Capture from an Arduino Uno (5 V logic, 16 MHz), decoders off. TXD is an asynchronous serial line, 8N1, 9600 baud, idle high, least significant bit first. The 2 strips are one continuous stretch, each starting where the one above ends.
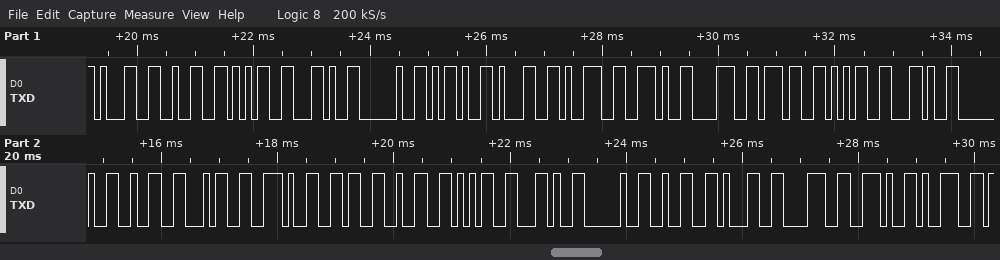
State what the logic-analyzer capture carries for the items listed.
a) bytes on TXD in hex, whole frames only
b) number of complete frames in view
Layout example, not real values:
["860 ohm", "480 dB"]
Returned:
["31 32 35 2C 20 2D 31 39 2E 38 37 35 2C 20 32 34 2E 36 32 35 2C 20 32 31 38 2E 39", "27"]
